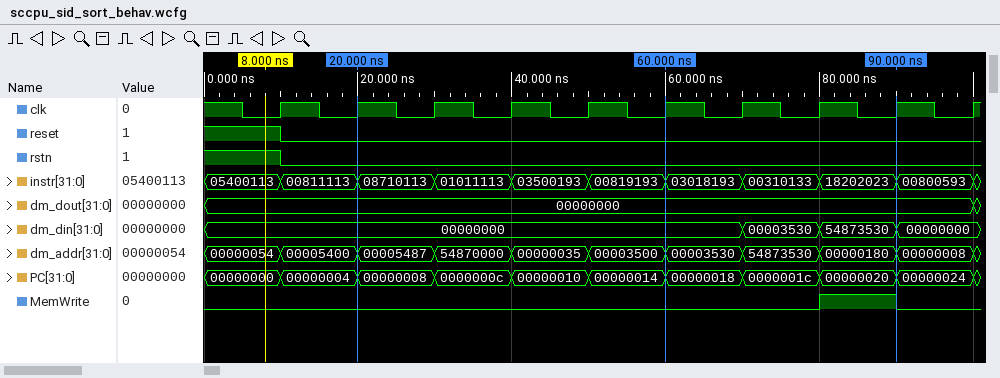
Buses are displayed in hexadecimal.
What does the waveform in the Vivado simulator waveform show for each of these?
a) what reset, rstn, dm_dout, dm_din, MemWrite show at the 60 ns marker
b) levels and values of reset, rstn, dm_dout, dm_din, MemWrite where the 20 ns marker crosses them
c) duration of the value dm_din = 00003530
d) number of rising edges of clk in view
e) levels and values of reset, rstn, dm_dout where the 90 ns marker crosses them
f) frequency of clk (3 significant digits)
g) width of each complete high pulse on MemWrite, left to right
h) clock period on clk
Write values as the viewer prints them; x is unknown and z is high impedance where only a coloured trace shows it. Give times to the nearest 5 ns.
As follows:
reset=0, rstn=0, dm_dout=00000000, dm_din=00000000, MemWrite=0
reset=0, rstn=0, dm_dout=00000000, dm_din=00000000, MemWrite=0
10 ns
10
reset=0, rstn=0, dm_dout=00000000
100 MHz
10 ns
10 ns
